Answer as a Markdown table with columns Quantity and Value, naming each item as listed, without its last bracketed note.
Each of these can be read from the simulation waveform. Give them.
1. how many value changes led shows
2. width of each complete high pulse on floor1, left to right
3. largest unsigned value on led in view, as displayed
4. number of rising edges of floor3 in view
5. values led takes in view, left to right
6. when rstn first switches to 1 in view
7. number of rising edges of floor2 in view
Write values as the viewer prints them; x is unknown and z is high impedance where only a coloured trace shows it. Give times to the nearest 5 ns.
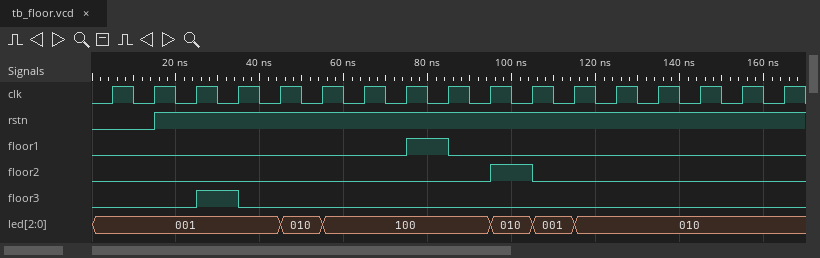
| Quantity | Value |
|---|---|
| how many value changes led shows | 5 |
| width of each complete high pulse on floor1, left to right | 10 ns |
| largest unsigned value on led in view, as displayed | 100 |
| number of rising edges of floor3 in view | 1 |
| values led takes in view, left to right | 001, 010, 100, 010, 001, 010 |
| when rstn first switches to 1 in view | 15 ns |
| number of rising edges of floor2 in view | 1 |
